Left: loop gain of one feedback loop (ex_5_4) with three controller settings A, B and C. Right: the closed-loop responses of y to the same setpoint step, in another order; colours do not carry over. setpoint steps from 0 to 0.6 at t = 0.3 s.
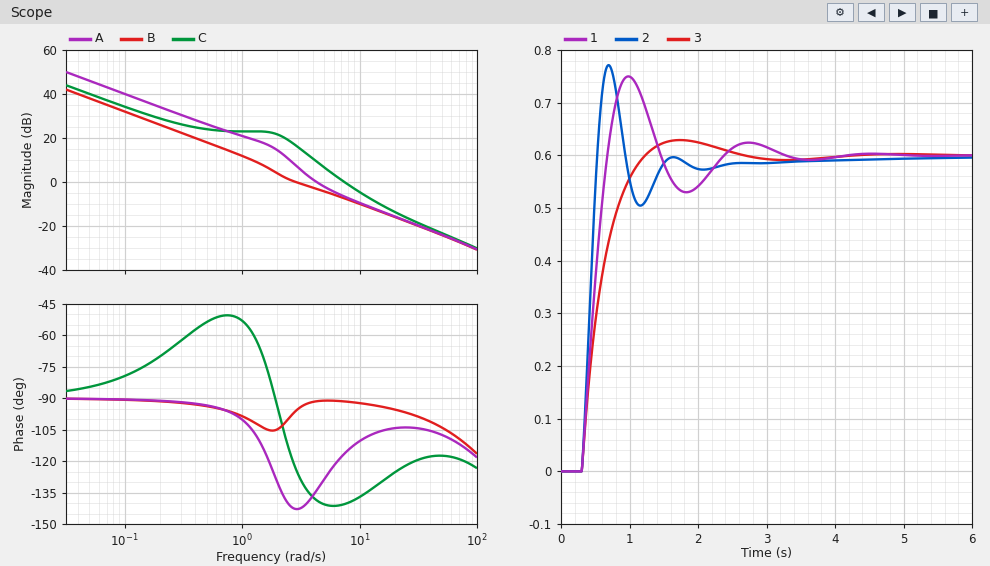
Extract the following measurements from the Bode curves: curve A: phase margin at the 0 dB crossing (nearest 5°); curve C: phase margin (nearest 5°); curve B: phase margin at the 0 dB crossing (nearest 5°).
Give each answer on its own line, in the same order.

45°
40°
85°
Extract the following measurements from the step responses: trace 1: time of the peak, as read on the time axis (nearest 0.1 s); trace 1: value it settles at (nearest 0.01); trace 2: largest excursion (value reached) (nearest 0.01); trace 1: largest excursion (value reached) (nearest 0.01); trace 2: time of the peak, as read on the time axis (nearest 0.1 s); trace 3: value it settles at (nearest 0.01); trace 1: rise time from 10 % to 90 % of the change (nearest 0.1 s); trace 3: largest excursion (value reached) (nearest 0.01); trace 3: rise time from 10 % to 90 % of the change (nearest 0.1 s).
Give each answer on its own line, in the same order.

1.0 s
0.60
0.77
0.75
0.7 s
0.60
0.3 s
0.63
0.6 s
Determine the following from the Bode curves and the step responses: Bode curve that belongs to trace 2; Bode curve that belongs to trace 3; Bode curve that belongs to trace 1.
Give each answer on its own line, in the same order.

C
B
A
